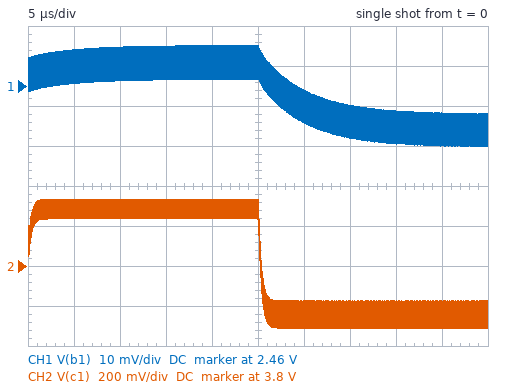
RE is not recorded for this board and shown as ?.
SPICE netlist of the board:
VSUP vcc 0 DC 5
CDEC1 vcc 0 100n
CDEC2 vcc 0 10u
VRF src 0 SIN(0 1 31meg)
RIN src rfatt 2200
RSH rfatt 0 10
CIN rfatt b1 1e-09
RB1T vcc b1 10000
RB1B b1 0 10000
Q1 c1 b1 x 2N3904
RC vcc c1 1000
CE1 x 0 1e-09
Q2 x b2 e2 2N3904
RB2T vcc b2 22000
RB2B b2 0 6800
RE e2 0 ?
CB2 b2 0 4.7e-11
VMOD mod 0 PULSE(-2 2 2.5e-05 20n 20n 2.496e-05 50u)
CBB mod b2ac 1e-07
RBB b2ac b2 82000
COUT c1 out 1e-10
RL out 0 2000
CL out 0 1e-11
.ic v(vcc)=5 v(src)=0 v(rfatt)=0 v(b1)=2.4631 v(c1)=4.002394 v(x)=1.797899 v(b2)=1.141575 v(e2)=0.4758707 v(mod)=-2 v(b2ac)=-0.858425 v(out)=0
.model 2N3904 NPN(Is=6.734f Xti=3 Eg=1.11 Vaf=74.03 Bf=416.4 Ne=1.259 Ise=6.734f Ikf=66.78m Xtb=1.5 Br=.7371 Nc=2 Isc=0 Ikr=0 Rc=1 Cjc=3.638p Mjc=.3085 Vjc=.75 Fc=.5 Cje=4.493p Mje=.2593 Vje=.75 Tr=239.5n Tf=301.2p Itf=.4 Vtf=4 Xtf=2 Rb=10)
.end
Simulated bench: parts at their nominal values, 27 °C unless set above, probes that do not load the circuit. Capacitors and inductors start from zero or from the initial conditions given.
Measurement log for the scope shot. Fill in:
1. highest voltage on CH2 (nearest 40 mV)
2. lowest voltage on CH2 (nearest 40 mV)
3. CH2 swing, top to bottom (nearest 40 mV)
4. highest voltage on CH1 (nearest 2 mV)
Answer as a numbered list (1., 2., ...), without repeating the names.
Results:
1. 4.12 V
2. 3.48 V
3. 640 mV
4. 2.470 V
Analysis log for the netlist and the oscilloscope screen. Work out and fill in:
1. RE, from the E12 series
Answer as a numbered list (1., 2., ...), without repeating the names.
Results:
1. 390 Ω
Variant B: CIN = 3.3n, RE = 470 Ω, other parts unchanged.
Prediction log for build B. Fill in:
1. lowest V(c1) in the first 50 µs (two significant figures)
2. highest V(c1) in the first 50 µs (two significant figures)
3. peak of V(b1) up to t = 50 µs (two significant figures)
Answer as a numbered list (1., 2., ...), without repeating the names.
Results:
1. 3.7 V
2. 4.3 V
3. 2.5 V
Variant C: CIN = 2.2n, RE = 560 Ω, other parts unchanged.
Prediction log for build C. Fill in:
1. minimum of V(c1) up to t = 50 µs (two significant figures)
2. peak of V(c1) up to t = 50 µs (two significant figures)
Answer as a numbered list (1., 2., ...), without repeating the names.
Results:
1. 3.9 V
2. 4.4 V
